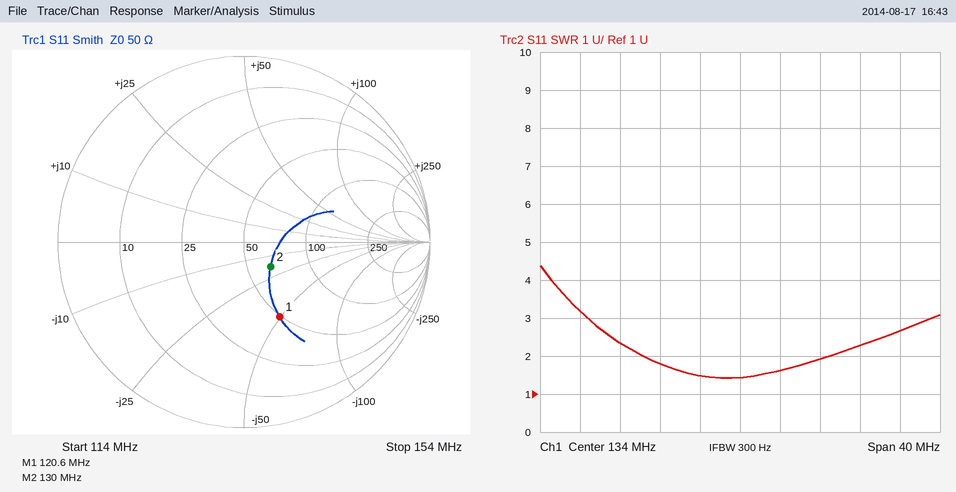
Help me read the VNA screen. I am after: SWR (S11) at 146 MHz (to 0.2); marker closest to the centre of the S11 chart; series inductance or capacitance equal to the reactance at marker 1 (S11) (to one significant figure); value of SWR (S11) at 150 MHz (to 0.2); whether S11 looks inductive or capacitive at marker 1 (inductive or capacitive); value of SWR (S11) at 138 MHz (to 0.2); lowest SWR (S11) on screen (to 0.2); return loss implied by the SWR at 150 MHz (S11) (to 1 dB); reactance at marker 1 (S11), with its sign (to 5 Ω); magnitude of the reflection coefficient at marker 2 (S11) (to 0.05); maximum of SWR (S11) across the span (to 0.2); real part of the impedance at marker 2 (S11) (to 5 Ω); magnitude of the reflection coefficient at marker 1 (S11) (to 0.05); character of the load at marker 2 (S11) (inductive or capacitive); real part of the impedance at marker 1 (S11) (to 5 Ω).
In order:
2.2
marker 2
30 pF
2.6
capacitive
1.6
1.4
7 dB
-50 Ω
0.20
4.4
65 Ω
0.45
capacitive
50 Ω
